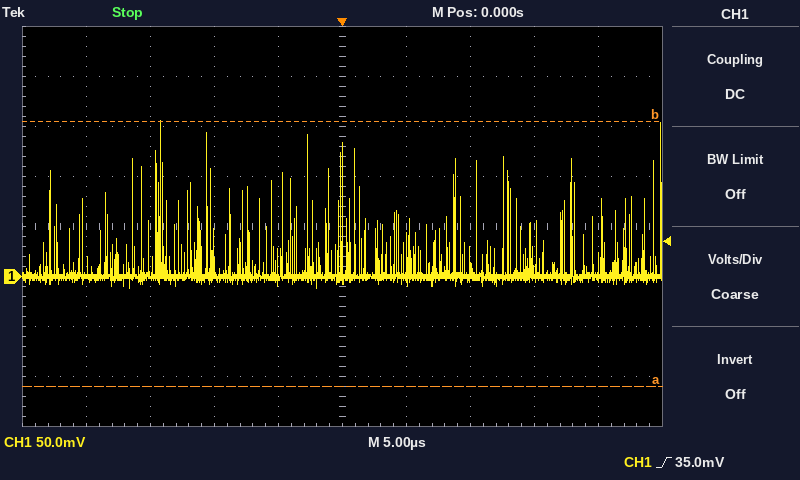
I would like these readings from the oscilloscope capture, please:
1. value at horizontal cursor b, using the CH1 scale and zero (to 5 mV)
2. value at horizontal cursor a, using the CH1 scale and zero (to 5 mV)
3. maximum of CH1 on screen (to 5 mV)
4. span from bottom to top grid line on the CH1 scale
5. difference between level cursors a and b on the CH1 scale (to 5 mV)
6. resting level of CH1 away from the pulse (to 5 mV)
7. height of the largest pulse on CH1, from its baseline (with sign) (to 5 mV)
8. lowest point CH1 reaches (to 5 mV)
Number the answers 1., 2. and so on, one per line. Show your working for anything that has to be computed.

1. 155 mV
2. -110 mV
3. 155 mV
4. 400 mV
5. 265 mV
6. 0 mV
7. 155 mV − (0 mV) = +155 mV
8. -10 mV
